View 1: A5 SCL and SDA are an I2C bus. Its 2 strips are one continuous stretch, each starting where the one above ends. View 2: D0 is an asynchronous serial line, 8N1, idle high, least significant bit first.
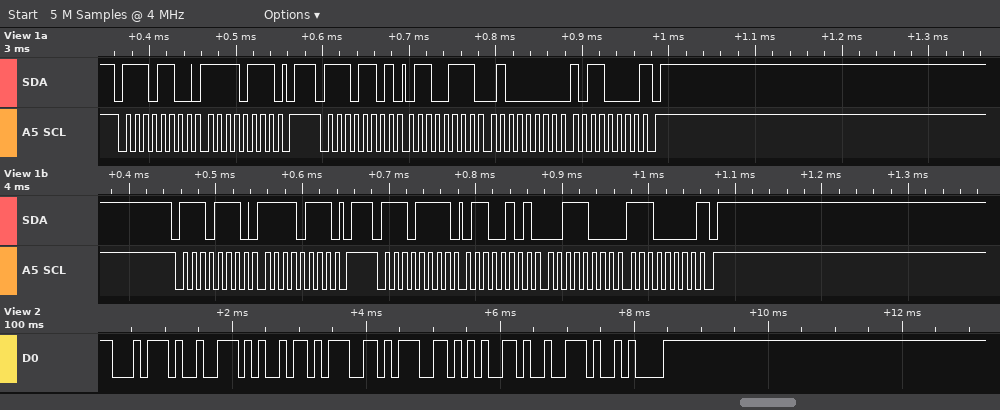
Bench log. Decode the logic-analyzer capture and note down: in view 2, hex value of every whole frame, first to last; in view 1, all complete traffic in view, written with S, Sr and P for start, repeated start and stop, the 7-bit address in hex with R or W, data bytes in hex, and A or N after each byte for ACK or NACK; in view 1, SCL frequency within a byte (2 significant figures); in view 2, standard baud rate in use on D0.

74 72 69 67 67 65 72 0A
S 76W A F7 A P S 76R A 67 A 40 A B0 N P S 77W A F7 A P S 77R A 65 A 38 A E0 N P
100 kHz
9600 baud
